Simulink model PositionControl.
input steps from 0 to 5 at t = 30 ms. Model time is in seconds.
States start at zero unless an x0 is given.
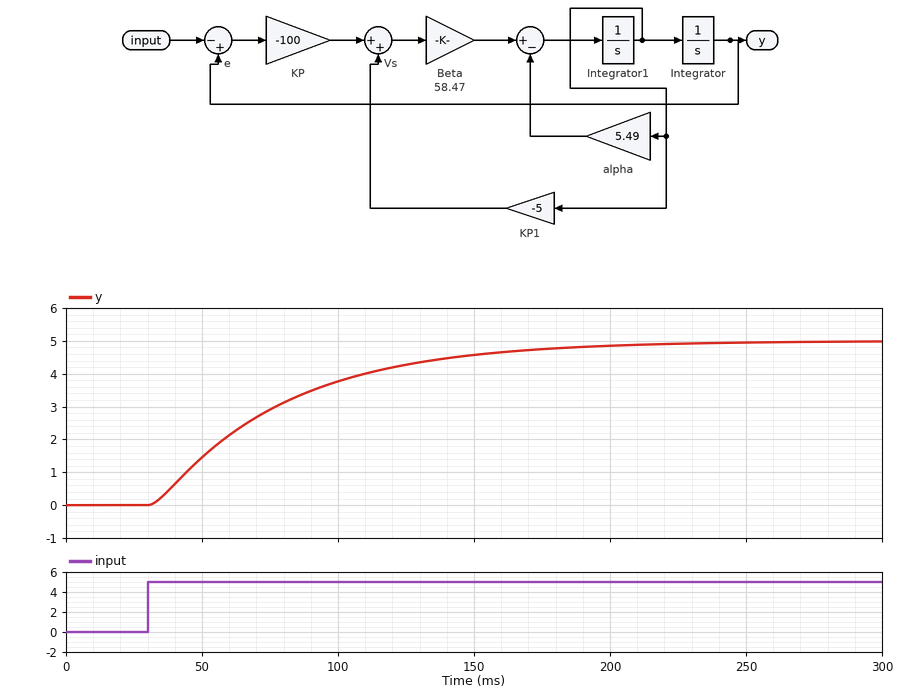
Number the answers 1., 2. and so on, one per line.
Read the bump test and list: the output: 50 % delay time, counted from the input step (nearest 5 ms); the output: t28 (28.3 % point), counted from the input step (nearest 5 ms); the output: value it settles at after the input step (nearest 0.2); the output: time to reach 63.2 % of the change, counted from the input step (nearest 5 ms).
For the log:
1. 35 ms
2. 20 ms
3. 5.0
4. 50 ms
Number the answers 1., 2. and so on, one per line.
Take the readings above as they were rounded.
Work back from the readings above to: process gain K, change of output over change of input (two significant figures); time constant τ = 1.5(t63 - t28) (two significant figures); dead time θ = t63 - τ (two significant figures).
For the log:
1. 1.0
2. 45 ms
3. 5.0 ms
